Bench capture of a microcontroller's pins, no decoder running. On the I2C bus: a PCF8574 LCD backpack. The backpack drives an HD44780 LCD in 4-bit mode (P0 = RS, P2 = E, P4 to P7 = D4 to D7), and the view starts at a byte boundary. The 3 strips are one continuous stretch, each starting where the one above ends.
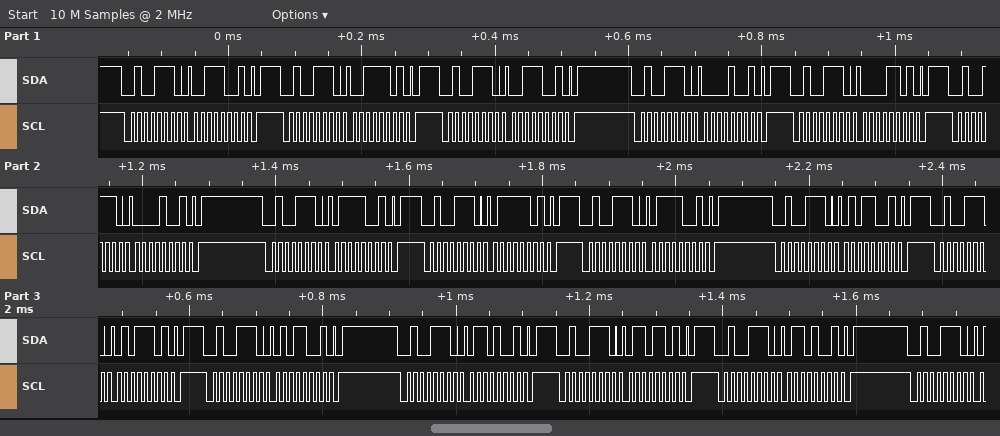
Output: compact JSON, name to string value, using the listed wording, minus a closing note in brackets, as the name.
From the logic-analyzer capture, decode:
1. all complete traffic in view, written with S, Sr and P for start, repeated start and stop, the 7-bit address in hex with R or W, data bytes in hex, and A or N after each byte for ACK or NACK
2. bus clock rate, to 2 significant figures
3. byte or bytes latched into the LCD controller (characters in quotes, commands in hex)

{"all complete traffic in view, written with S, Sr and P for start, repeated start and stop, the 7-bit address in hex with R or W, data bytes in hex, and A or N after each byte for ACK or NACK": "S 27W A 39 A P S 27W A 3D A P S 27W A 39 A P S 27W A 09 A P S 27W A 0D A P S 27W A 09 A P S 27W A 79 A P S 27W A 7D A P S 27W A 79 A P S 27W A 59 A P S 27W A 5D A P S 27W A 59 A P S 27W A 69 A P S 27W A 6D A P S 27W A 69 A P S 27W A", "bus clock rate, to 2 significant figures": "100 kHz", "byte or bytes latched into the LCD controller": "'0' 'u'"}
